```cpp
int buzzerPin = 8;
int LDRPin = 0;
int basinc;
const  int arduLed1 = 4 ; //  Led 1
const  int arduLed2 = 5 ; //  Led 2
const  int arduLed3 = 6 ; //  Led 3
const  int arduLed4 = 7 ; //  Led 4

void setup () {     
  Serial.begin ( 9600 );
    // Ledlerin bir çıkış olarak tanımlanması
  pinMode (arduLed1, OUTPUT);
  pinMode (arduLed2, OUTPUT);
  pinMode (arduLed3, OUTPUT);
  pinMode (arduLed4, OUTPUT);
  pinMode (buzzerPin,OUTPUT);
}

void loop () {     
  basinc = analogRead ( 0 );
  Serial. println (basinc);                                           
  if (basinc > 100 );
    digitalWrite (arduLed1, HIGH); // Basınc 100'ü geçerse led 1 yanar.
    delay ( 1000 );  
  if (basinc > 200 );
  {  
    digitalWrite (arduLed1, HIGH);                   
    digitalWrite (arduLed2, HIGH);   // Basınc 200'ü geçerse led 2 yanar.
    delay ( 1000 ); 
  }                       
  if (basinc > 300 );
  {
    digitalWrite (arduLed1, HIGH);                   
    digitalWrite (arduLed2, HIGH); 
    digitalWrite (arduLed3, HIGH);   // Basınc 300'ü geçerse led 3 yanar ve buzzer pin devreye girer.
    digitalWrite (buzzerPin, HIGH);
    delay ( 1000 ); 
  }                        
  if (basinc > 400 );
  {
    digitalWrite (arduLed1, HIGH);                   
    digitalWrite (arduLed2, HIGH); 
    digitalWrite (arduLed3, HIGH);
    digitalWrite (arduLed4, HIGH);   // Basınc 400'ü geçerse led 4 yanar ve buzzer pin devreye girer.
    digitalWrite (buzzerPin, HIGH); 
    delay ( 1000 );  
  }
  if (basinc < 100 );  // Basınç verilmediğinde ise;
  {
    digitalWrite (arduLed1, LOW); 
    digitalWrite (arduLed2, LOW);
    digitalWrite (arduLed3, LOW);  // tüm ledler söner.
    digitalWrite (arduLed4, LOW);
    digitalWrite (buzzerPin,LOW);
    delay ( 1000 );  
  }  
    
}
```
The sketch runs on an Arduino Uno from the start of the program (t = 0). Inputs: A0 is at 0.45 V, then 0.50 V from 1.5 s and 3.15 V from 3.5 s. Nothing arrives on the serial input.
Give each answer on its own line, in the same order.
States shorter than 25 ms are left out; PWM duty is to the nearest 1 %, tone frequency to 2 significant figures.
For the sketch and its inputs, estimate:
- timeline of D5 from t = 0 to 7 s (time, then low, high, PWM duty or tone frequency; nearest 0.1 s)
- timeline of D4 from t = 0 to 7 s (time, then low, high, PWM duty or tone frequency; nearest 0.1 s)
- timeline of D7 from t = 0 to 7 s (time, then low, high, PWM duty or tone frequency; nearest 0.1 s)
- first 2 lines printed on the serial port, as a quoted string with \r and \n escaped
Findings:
0 s low; 1 s high; 4 s low; 6 s high
0 s high; 4 s low; 5 s high
0 s low; 3 s high; 4 s low
"92\r\n645\r\n"
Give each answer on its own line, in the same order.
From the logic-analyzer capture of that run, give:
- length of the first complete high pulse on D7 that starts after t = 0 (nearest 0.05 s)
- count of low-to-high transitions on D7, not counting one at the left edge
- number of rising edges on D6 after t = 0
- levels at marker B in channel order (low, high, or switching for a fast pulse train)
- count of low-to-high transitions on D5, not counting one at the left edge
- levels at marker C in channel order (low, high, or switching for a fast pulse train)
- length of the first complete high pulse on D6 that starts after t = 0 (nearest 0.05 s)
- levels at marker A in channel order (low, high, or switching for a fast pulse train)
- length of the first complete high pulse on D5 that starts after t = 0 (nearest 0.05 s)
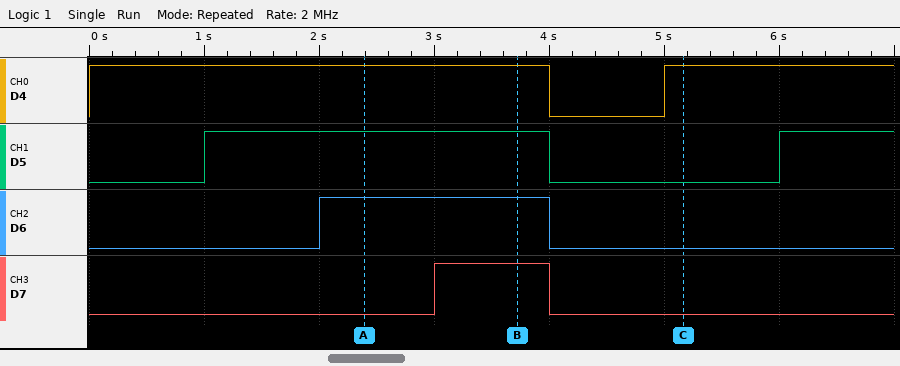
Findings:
1.00 s
1
1
D4 high, D5 high, D6 high, D7 high
2
D4 high, D5 low, D6 low, D7 low
2.00 s
D4 high, D5 high, D6 high, D7 low
3.00 s
